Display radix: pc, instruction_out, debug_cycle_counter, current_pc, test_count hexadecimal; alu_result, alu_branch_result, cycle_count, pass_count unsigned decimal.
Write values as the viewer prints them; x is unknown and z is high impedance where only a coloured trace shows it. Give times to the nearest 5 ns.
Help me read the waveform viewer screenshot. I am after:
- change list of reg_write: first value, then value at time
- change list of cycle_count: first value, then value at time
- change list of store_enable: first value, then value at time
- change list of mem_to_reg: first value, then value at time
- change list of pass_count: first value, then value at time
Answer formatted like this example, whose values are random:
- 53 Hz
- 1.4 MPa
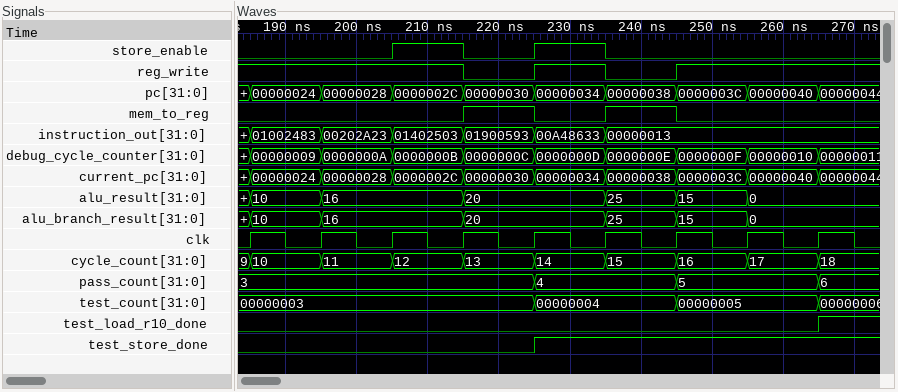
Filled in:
- 1, 0 at 215 ns, 1 at 225 ns, 0 at 235 ns, 1 at 245 ns
- 9, 10 at 185 ns, 11 at 195 ns, 12 at 205 ns, 13 at 215 ns, 14 at 225 ns, 15 at 235 ns, 16 at 245 ns, 17 at 255 ns, 18 at 265 ns
- 0, 1 at 205 ns, 0 at 215 ns, 1 at 225 ns, 0 at 235 ns
- 0, 1 at 215 ns, 0 at 225 ns, 1 at 235 ns, 0 at 245 ns
- 3, 4 at 225 ns, 5 at 245 ns, 6 at 265 ns
